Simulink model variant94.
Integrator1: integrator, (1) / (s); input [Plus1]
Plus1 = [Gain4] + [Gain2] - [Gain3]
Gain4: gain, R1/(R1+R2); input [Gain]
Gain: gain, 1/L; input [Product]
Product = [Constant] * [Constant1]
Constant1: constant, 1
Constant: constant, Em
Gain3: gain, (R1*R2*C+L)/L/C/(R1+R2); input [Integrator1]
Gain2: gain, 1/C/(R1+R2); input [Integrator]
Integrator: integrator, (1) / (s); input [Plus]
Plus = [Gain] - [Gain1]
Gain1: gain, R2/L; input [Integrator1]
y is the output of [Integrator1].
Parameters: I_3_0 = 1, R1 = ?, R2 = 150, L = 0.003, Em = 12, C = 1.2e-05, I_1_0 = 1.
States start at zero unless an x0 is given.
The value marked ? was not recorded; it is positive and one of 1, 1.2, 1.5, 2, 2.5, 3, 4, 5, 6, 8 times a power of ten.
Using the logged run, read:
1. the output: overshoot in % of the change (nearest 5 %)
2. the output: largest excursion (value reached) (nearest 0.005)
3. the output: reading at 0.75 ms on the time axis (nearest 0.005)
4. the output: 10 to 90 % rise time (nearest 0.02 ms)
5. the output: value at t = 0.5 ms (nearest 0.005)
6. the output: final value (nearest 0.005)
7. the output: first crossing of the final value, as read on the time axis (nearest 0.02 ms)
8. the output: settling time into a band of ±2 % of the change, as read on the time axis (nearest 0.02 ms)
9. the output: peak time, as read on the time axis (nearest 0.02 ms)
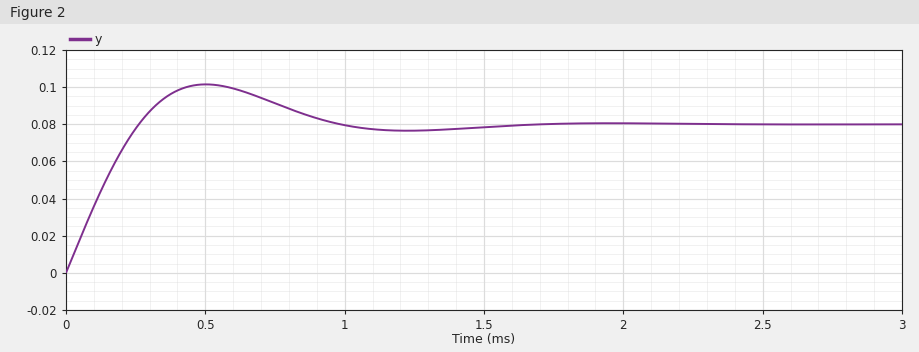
25 %
0.100
0.090
0.20 ms
0.100
0.080
0.26 ms
1.50 ms
0.50 ms
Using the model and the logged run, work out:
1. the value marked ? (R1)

15
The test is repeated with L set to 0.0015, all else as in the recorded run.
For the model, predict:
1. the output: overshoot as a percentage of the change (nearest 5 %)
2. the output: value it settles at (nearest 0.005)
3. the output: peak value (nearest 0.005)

20 %
0.080
0.095
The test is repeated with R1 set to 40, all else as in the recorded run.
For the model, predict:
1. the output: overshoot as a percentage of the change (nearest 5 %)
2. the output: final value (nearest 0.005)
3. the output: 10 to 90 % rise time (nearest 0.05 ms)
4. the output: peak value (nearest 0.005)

10 %
0.080
0.15 ms
0.085
